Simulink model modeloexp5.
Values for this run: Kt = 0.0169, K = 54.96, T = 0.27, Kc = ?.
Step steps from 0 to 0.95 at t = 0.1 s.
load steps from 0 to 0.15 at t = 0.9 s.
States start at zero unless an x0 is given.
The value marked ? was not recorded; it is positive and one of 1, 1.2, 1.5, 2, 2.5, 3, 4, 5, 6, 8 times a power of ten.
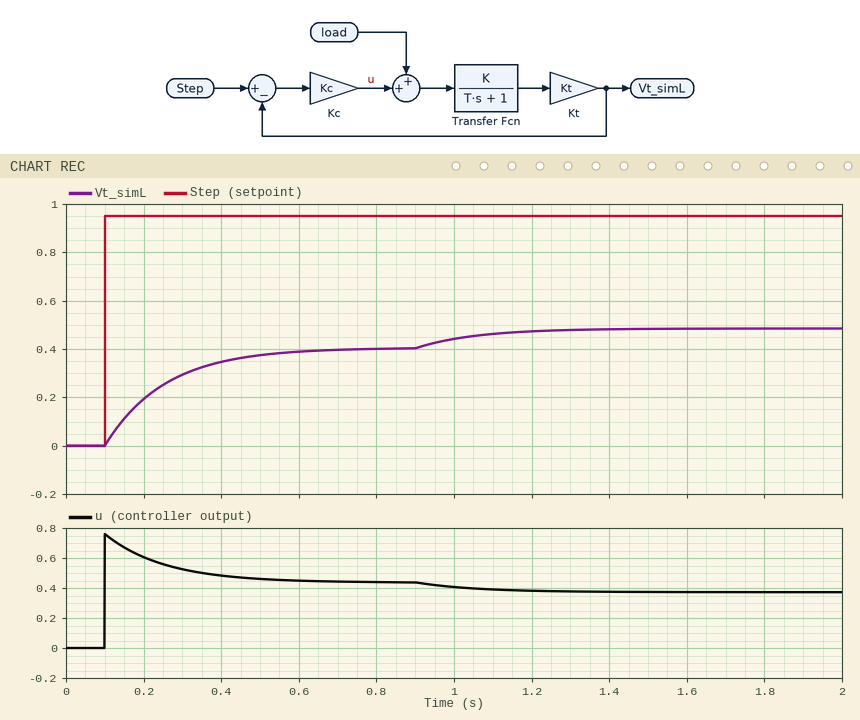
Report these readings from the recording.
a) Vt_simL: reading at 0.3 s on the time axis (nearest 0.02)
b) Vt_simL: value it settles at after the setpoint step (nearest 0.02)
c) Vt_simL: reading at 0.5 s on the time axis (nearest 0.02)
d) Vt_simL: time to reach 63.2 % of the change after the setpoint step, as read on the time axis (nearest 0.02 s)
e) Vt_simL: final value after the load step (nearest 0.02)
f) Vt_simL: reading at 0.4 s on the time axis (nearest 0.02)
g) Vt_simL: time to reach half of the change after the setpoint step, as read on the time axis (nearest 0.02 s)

0.30
0.40
0.38
0.26 s
0.48
0.34
0.20 s
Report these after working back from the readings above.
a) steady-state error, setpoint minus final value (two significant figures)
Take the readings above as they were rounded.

0.55
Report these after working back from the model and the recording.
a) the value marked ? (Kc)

0.8
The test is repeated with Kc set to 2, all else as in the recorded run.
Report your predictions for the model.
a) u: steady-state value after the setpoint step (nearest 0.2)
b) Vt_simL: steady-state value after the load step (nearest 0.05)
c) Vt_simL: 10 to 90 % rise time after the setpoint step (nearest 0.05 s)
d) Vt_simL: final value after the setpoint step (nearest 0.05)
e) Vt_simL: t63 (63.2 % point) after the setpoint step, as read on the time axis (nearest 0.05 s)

0.6
0.65
0.20 s
0.60
0.20 s
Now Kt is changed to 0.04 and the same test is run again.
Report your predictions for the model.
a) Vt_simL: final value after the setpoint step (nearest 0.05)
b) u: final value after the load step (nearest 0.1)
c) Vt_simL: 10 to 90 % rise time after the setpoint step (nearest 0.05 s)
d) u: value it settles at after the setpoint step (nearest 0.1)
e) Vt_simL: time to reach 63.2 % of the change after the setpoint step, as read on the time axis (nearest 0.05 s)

0.60
0.2
0.20 s
0.3
0.20 s
